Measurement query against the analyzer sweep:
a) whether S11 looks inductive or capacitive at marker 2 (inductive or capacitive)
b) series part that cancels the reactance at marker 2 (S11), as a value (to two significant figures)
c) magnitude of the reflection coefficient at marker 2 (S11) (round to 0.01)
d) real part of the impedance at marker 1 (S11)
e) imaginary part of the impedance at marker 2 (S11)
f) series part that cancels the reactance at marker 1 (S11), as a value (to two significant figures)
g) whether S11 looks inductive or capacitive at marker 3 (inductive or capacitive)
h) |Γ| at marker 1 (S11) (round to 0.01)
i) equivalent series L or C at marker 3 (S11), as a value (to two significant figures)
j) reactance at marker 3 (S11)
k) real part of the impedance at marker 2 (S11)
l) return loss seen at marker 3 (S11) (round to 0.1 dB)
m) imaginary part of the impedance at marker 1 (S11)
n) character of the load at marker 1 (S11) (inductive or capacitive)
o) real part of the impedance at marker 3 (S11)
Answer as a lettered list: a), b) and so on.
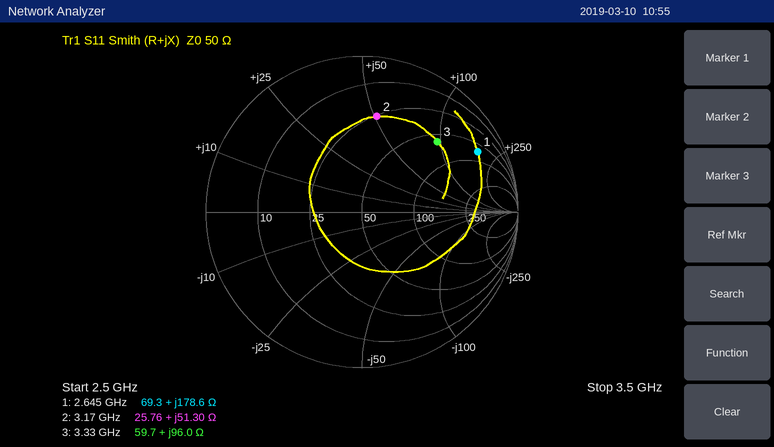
a) inductive
b) 980 fF
c) 0.62
d) 69.3 Ω
e) +51.30 Ω
f) 340 fF
g) inductive
h) 0.84
i) 4.6 nH
j) +96.0 Ω
k) 25.76 Ω
l) 3.6 dB
m) +178.6 Ω
n) inductive
o) 59.7 Ω
